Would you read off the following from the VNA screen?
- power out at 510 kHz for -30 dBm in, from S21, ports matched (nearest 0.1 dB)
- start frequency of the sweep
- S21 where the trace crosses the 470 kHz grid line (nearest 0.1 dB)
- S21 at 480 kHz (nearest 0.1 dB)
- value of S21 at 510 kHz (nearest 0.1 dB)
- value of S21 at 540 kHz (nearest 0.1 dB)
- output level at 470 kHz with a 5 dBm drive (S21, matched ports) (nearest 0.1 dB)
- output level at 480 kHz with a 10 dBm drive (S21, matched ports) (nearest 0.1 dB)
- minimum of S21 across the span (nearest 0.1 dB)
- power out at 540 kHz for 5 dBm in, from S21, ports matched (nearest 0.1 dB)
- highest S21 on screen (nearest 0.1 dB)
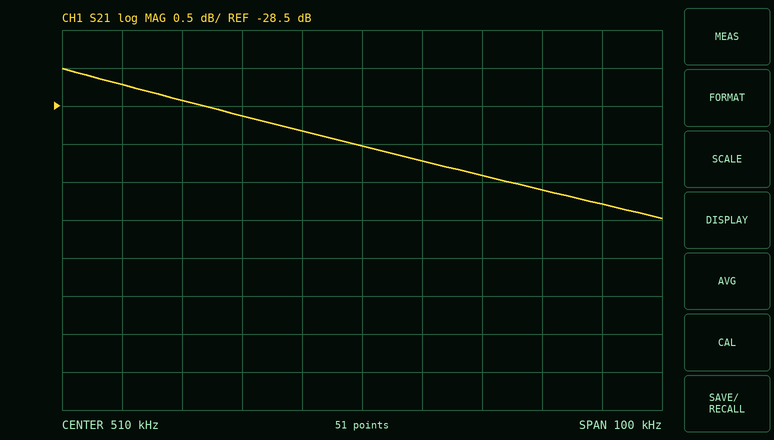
-59.0 dBm
460 kHz
-28.2 dB
-28.4 dB
-29.0 dB
-29.6 dB
-23.2 dBm
-18.4 dBm
-30.0 dB
-24.6 dBm
-28.0 dB
